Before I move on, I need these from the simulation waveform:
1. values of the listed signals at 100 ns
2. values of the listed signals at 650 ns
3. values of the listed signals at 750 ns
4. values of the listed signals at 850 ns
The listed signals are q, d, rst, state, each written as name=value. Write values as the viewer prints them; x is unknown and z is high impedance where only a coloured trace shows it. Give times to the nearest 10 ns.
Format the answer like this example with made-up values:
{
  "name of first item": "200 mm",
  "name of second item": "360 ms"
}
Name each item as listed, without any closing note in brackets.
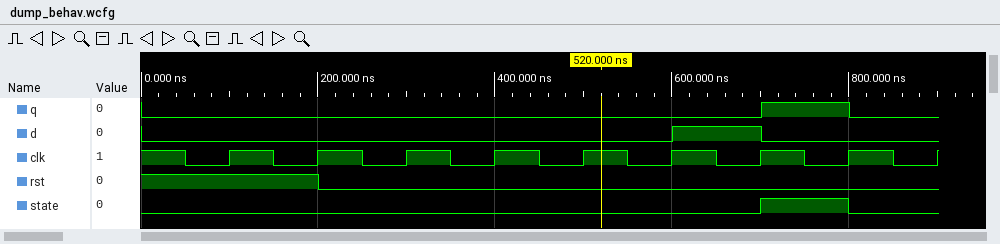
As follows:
{
  "values of the listed signals at 100 ns": "q=0, d=0, rst=1, state=0",
  "values of the listed signals at 650 ns": "q=0, d=1, rst=0, state=0",
  "values of the listed signals at 750 ns": "q=1, d=0, rst=0, state=1",
  "values of the listed signals at 850 ns": "q=0, d=0, rst=0, state=0"
}
